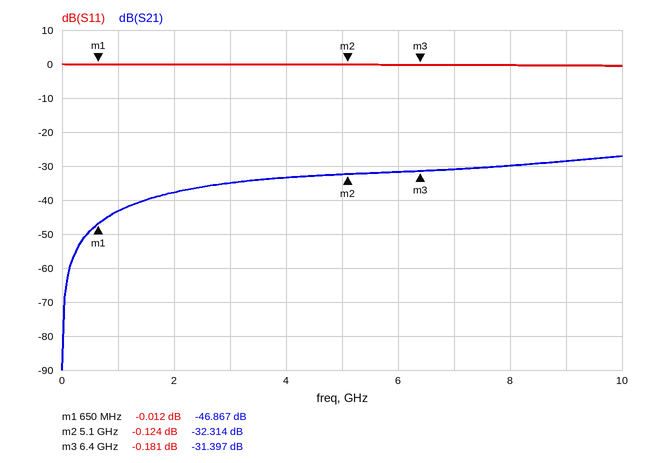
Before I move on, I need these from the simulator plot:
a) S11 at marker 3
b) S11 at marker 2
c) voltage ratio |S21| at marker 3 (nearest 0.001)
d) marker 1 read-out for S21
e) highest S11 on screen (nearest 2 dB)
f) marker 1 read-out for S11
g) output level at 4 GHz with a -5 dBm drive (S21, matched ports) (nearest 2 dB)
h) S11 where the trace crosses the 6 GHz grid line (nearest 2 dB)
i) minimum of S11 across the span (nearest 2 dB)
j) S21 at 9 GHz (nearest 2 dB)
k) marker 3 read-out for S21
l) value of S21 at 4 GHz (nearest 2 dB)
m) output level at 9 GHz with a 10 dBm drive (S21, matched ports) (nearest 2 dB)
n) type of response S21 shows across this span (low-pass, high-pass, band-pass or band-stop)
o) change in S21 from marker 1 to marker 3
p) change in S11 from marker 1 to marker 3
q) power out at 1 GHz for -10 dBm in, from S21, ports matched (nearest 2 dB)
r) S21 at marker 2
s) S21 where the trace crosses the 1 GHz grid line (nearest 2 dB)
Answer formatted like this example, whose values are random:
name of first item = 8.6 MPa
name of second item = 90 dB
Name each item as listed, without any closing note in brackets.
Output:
S11 at marker 3 = -0.181 dB
S11 at marker 2 = -0.124 dB
voltage ratio |S21| at marker 3 = 0.027
marker 1 read-out for S21 = -46.867 dB
highest S11 on screen = 0 dB
marker 1 read-out for S11 = -0.012 dB
output level at 4 GHz with a -5 dBm drive (S21, matched ports) = -38 dBm
S11 where the trace crosses the 6 GHz grid line = 0 dB
minimum of S11 across the span = 0 dB
S21 at 9 GHz = -28 dB
marker 3 read-out for S21 = -31.397 dB
value of S21 at 4 GHz = -34 dB
output level at 9 GHz with a 10 dBm drive (S21, matched ports) = -18 dBm
type of response S21 shows across this span = high-pass
change in S21 from marker 1 to marker 3 = 15.470 dB
change in S11 from marker 1 to marker 3 = -0.169 dB
power out at 1 GHz for -10 dBm in, from S21, ports matched = -54 dBm
S21 at marker 2 = -32.314 dB
S21 where the trace crosses the 1 GHz grid line = -44 dB
